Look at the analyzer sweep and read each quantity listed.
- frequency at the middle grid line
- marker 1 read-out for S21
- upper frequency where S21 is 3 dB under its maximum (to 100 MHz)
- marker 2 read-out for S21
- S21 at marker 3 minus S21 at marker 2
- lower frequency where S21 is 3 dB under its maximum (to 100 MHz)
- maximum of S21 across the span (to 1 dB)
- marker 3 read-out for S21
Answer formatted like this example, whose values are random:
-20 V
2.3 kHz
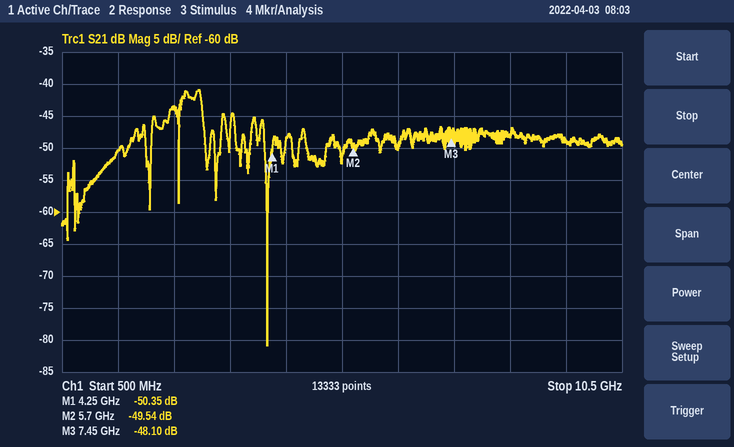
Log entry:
5.5 GHz
-50.35 dB
3.0 GHz
-49.54 dB
1.44 dB
2.6 GHz
-41 dB
-48.10 dB
